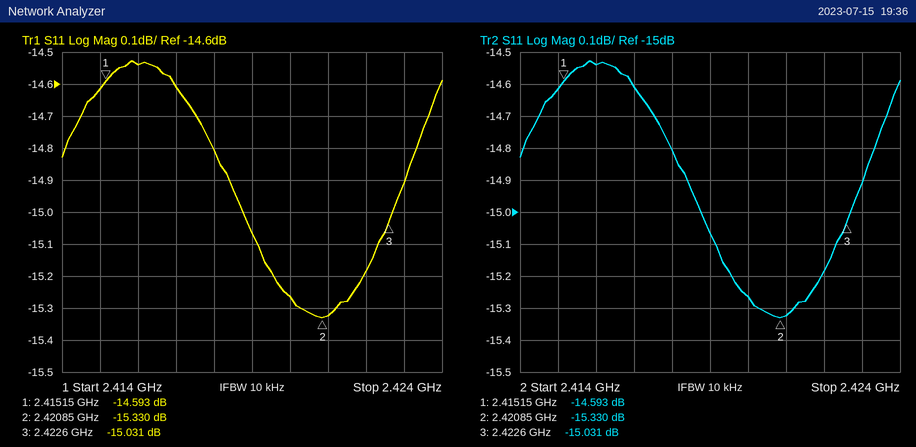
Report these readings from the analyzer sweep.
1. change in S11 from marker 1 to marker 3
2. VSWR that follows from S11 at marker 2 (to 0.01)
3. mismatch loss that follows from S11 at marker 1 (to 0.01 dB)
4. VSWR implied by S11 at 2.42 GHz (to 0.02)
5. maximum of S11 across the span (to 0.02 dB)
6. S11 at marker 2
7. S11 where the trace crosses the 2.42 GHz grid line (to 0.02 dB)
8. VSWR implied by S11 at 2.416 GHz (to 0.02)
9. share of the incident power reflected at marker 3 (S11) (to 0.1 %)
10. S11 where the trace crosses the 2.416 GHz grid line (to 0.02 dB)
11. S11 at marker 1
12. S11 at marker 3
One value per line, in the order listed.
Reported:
-0.438 dB
1.41
0.15 dB
1.42
-14.52 dB
-15.330 dB
-15.26 dB
1.46
3.1 %
-14.54 dB
-14.593 dB
-15.031 dB
